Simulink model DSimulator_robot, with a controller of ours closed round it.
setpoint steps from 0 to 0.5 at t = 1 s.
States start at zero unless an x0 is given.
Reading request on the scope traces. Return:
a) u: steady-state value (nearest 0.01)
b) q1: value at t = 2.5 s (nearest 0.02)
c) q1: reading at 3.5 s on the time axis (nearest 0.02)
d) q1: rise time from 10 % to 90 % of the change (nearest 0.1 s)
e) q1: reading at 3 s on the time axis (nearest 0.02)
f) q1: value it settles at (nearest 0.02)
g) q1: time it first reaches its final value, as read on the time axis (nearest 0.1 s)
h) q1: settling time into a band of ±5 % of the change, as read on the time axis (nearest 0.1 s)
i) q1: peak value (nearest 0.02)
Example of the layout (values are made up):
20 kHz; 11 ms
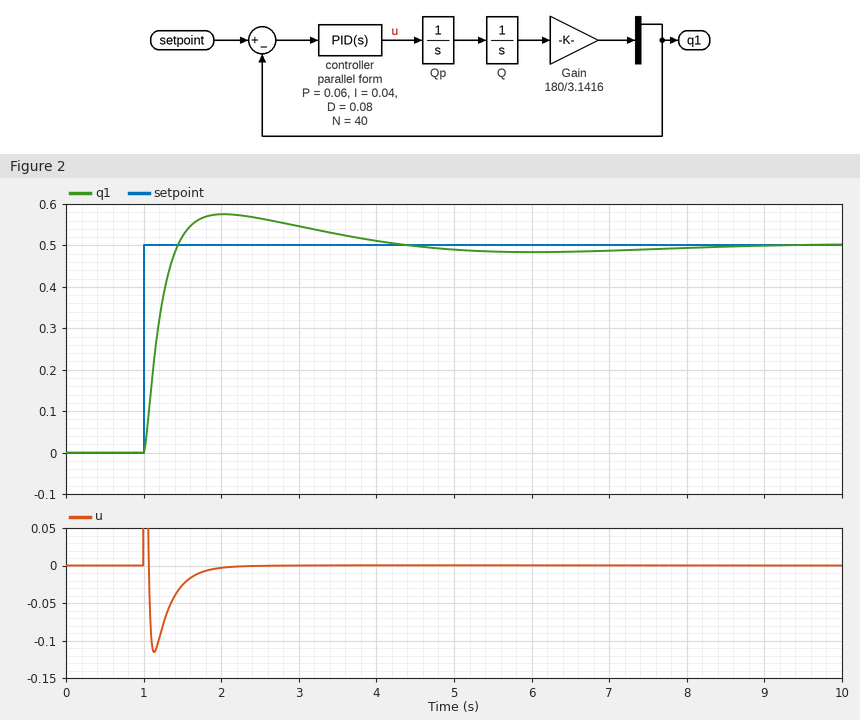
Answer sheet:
0.00; 0.56; 0.52; 0.3 s; 0.54; 0.50; 1.4 s; 3.6 s; 0.58
